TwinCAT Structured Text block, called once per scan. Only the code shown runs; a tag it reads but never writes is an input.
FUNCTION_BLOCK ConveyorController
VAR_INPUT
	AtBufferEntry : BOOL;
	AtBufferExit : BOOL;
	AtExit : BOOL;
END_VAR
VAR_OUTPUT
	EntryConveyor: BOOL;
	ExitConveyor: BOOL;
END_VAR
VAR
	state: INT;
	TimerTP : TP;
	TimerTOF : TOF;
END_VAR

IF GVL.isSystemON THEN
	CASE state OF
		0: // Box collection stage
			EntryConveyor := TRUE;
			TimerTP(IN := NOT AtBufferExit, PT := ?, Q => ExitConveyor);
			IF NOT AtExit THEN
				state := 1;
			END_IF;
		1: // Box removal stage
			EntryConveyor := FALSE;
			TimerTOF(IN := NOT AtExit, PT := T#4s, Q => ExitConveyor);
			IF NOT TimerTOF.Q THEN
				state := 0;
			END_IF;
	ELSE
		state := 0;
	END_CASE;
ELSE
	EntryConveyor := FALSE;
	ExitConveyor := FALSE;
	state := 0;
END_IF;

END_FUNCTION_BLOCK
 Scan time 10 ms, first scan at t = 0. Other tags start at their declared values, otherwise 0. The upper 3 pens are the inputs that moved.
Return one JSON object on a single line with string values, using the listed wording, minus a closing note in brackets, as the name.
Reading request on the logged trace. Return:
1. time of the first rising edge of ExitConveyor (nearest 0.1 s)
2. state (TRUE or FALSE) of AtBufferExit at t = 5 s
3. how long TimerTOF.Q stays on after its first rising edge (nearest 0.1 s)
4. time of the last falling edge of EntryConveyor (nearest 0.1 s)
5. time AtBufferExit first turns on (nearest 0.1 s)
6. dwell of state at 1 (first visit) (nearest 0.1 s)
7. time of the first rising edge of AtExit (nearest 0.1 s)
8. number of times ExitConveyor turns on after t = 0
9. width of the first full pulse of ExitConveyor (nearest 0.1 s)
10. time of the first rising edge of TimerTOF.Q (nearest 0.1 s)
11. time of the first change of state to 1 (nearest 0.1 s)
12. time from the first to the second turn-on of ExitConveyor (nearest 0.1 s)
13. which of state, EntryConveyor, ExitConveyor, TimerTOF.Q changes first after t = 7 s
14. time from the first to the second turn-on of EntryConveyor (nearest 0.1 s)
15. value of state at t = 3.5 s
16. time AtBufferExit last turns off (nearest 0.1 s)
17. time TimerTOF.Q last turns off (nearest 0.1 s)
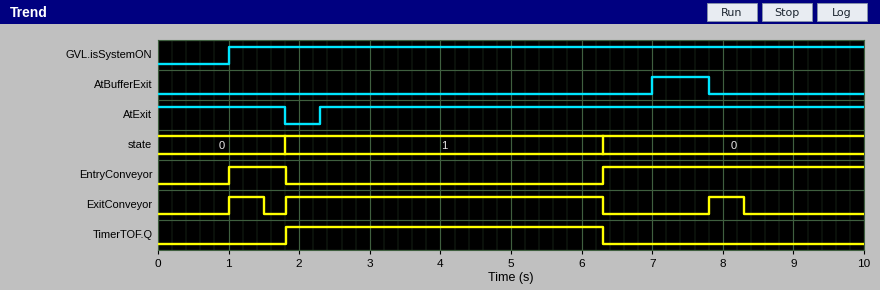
{"time of the first rising edge of ExitConveyor": "1.0 s", "state (TRUE or FALSE) of AtBufferExit at t = 5 s": "FALSE", "how long TimerTOF.Q stays on after its first rising edge": "4.5 s", "time of the last falling edge of EntryConveyor": "1.8 s", "time AtBufferExit first turns on": "7.0 s", "dwell of state at 1 (first visit)": "4.5 s", "time of the first rising edge of AtExit": "2.3 s", "number of times ExitConveyor turns on after t = 0": "3", "width of the first full pulse of ExitConveyor": "0.5 s", "time of the first rising edge of TimerTOF.Q": "1.8 s", "time of the first change of state to 1": "1.8 s", "time from the first to the second turn-on of ExitConveyor": "0.8 s", "which of state, EntryConveyor, ExitConveyor, TimerTOF.Q changes first after t = 7 s": "ExitConveyor", "time from the first to the second turn-on of EntryConveyor": "5.3 s", "value of state at t = 3.5 s": "1", "time AtBufferExit last turns off": "7.8 s", "time TimerTOF.Q last turns off": "6.3 s"}
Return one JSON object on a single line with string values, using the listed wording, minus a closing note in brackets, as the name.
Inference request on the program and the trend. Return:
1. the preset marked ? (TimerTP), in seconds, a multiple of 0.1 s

{"the preset marked ? (TimerTP), in seconds, a multiple of 0.1 s": "0.5 s"}
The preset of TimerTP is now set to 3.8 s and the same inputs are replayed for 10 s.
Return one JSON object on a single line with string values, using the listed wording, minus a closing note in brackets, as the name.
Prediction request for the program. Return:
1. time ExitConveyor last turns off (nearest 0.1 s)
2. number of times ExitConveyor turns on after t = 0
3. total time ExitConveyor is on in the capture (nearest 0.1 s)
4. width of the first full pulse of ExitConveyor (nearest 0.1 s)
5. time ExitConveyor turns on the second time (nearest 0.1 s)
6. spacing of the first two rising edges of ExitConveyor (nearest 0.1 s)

{"time ExitConveyor last turns off": "6.3 s", "number of times ExitConveyor turns on after t = 0": "2", "total time ExitConveyor is on in the capture": "7.5 s", "width of the first full pulse of ExitConveyor": "5.3 s", "time ExitConveyor turns on the second time": "7.8 s", "spacing of the first two rising edges of ExitConveyor": "6.8 s"}
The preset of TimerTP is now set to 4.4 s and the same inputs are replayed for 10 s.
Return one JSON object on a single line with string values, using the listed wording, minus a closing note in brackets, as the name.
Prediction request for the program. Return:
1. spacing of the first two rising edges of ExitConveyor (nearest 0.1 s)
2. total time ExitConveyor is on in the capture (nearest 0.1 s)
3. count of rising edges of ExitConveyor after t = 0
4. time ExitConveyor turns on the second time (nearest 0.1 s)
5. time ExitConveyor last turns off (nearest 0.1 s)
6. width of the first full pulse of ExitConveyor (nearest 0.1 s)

{"spacing of the first two rising edges of ExitConveyor": "6.8 s", "total time ExitConveyor is on in the capture": "7.5 s", "count of rising edges of ExitConveyor after t = 0": "2", "time ExitConveyor turns on the second time": "7.8 s", "time ExitConveyor last turns off": "6.3 s", "width of the first full pulse of ExitConveyor": "5.3 s"}
